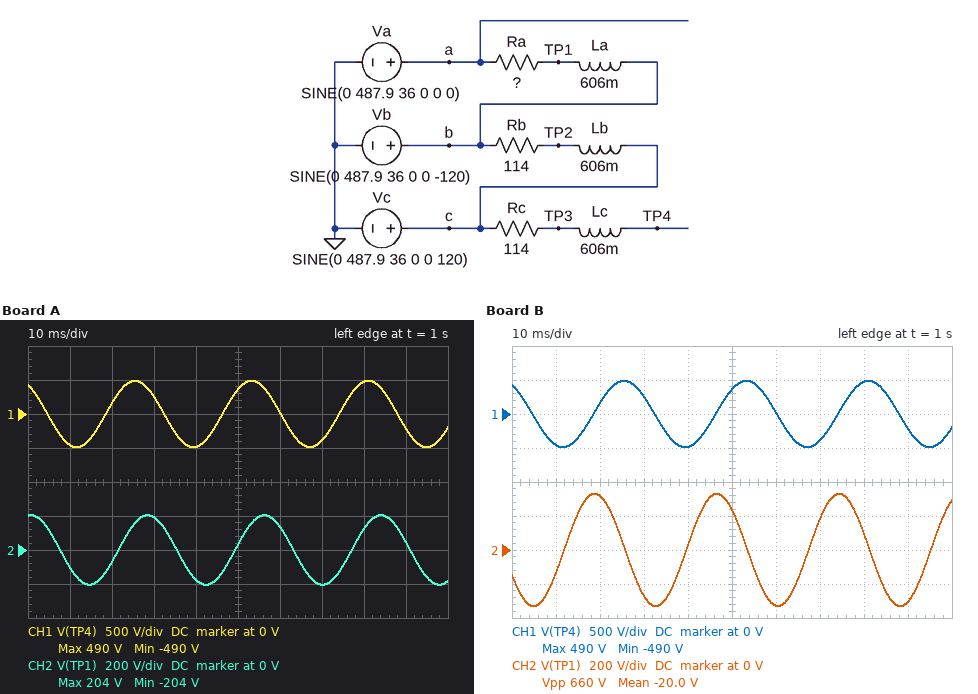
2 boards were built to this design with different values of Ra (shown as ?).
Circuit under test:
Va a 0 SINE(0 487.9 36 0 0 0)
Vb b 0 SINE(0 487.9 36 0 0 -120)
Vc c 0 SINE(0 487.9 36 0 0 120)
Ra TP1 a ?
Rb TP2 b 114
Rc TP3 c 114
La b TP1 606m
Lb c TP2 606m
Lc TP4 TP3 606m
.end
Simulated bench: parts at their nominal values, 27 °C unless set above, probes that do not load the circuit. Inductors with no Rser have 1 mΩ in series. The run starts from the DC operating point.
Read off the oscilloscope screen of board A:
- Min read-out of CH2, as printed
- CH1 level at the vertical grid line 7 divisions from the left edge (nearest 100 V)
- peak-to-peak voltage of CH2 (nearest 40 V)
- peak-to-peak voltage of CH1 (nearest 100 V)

-204 V
-400 V
400 V
1.0 kV
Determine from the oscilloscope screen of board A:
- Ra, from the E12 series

100 Ω
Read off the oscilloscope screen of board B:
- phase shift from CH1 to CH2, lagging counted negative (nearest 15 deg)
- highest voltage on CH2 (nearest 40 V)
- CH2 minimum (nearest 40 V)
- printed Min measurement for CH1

90 deg
320 V
-320 V
-490 V
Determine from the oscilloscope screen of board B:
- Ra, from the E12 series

390 Ω
